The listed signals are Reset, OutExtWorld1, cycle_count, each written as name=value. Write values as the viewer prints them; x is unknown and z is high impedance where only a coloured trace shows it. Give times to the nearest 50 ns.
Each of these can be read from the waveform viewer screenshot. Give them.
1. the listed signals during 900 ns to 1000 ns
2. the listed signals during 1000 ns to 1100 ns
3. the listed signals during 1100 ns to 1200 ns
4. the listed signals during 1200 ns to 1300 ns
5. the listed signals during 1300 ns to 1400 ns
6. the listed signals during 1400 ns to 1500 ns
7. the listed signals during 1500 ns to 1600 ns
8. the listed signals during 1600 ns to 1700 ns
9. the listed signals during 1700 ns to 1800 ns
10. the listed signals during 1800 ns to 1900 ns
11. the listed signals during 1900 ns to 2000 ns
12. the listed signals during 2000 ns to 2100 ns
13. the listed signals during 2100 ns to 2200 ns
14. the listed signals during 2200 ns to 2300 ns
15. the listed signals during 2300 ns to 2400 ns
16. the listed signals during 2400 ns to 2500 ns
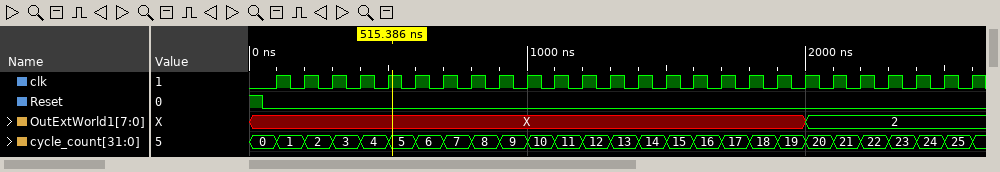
Reset=0, OutExtWorld1=X, cycle_count=9
Reset=0, OutExtWorld1=X, cycle_count=10
Reset=0, OutExtWorld1=X, cycle_count=11
Reset=0, OutExtWorld1=X, cycle_count=12
Reset=0, OutExtWorld1=X, cycle_count=13
Reset=0, OutExtWorld1=X, cycle_count=14
Reset=0, OutExtWorld1=X, cycle_count=15
Reset=0, OutExtWorld1=X, cycle_count=16
Reset=0, OutExtWorld1=X, cycle_count=17
Reset=0, OutExtWorld1=X, cycle_count=18
Reset=0, OutExtWorld1=X, cycle_count=19
Reset=0, OutExtWorld1=2, cycle_count=20
Reset=0, OutExtWorld1=2, cycle_count=21
Reset=0, OutExtWorld1=2, cycle_count=22
Reset=0, OutExtWorld1=2, cycle_count=23
Reset=0, OutExtWorld1=2, cycle_count=24
